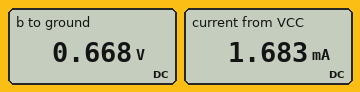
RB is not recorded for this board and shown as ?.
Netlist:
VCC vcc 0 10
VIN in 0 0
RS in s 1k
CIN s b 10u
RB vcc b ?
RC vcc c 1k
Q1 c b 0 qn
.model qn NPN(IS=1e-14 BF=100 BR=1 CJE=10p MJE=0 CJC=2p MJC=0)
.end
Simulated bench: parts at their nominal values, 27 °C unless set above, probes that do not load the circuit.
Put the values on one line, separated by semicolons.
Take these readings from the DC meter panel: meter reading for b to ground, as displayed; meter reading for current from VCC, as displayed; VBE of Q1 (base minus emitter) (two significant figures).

0.668 V; 1.683 mA; 670 mV
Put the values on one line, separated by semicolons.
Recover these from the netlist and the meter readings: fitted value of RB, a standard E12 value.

560 kΩ
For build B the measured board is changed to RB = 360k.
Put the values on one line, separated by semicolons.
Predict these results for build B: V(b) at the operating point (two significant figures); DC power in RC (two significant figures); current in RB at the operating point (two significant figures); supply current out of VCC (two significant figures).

680 mV; 6.7 mW; 26 µA; 2.6 mA
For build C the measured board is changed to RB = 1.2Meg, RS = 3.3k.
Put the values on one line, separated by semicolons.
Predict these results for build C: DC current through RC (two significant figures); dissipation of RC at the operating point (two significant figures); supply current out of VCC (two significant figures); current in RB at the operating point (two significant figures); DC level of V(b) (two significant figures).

780 µA; 610 µW; 790 µA; 7.8 µA; 650 mV
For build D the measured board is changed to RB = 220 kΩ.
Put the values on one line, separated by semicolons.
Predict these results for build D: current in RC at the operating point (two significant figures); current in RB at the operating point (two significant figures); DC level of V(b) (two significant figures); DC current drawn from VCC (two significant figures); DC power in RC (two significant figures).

4.2 mA; 42 µA; 690 mV; 4.3 mA; 18 mW
